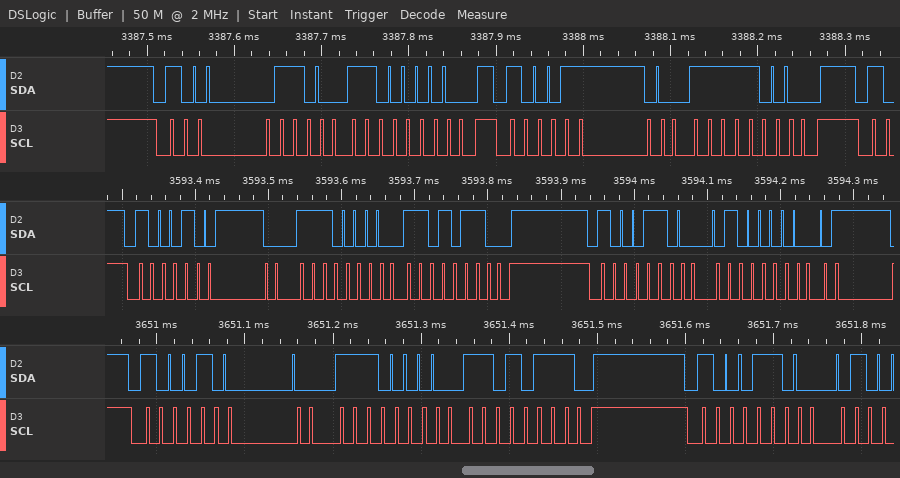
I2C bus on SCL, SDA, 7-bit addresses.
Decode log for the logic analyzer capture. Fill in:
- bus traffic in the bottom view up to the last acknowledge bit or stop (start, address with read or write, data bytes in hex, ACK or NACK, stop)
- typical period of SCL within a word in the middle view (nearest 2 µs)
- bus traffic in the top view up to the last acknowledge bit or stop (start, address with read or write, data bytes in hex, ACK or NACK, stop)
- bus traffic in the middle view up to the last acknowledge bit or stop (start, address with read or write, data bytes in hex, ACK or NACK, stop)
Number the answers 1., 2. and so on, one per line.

1. start, address 44 write ACK, E0 ACK, D7 ACK, stop, start, address 46 write ACK
2. 16 µs
3. start, address 46 write ACK, C0 ACK, stop, start, address 46 write ACK, F8 ACK, stop
4. start, address 44 write ACK, E0 ACK, D6 ACK, stop, start, address 46 write ACK, 40 ACK
